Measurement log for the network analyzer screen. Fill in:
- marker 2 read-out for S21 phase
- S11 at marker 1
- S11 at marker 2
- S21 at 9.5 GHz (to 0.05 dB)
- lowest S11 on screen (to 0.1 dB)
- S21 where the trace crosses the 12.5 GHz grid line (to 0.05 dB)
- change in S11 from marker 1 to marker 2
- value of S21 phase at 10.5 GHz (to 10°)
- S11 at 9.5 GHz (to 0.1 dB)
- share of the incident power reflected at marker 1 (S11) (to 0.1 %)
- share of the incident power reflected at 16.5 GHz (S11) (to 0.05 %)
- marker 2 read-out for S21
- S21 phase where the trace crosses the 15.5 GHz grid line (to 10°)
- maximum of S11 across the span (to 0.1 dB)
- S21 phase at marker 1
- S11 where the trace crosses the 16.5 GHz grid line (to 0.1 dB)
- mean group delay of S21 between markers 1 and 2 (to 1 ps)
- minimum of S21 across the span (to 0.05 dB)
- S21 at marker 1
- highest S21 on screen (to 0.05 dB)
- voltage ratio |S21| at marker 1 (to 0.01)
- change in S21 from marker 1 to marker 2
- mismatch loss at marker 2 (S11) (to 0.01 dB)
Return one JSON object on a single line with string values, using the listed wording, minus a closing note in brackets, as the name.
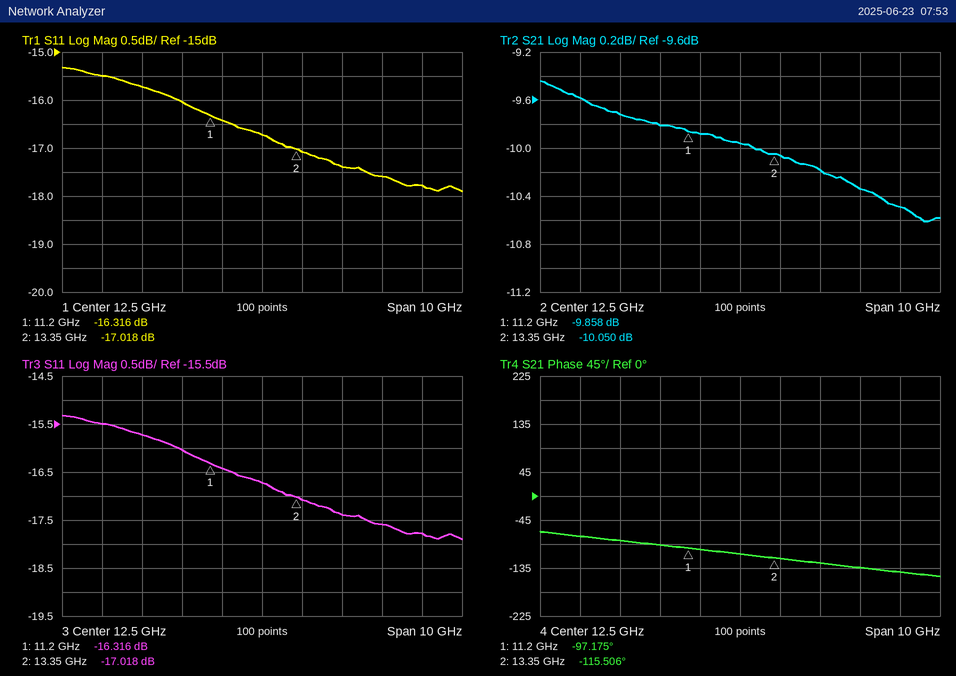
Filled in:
{"marker 2 read-out for S21 phase": "-115.506°", "S11 at marker 1": "-16.316 dB", "S11 at marker 2": "-17.018 dB", "S21 at 9.5 GHz": "-9.70 dB", "lowest S11 on screen": "-17.9 dB", "S21 where the trace crosses the 12.5 GHz grid line": "-9.95 dB", "change in S11 from marker 1 to marker 2": "-0.702 dB", "value of S21 phase at 10.5 GHz": "-90°", "S11 at 9.5 GHz": "-15.7 dB", "share of the incident power reflected at marker 1 (S11)": "2.3 %", "share of the incident power reflected at 16.5 GHz (S11)": "1.65 %", "marker 2 read-out for S21": "-10.050 dB", "S21 phase where the trace crosses the 15.5 GHz grid line": "-130°", "maximum of S11 across the span": "-15.3 dB", "S21 phase at marker 1": "-97.175°", "S11 where the trace crosses the 16.5 GHz grid line": "-17.8 dB", "mean group delay of S21 between markers 1 and 2": "24 ps", "minimum of S21 across the span": "-10.60 dB", "S21 at marker 1": "-9.858 dB", "highest S21 on screen": "-9.45 dB", "voltage ratio |S21| at marker 1": "0.32", "change in S21 from marker 1 to marker 2": "-0.192 dB", "mismatch loss at marker 2 (S11)": "0.09 dB"}
